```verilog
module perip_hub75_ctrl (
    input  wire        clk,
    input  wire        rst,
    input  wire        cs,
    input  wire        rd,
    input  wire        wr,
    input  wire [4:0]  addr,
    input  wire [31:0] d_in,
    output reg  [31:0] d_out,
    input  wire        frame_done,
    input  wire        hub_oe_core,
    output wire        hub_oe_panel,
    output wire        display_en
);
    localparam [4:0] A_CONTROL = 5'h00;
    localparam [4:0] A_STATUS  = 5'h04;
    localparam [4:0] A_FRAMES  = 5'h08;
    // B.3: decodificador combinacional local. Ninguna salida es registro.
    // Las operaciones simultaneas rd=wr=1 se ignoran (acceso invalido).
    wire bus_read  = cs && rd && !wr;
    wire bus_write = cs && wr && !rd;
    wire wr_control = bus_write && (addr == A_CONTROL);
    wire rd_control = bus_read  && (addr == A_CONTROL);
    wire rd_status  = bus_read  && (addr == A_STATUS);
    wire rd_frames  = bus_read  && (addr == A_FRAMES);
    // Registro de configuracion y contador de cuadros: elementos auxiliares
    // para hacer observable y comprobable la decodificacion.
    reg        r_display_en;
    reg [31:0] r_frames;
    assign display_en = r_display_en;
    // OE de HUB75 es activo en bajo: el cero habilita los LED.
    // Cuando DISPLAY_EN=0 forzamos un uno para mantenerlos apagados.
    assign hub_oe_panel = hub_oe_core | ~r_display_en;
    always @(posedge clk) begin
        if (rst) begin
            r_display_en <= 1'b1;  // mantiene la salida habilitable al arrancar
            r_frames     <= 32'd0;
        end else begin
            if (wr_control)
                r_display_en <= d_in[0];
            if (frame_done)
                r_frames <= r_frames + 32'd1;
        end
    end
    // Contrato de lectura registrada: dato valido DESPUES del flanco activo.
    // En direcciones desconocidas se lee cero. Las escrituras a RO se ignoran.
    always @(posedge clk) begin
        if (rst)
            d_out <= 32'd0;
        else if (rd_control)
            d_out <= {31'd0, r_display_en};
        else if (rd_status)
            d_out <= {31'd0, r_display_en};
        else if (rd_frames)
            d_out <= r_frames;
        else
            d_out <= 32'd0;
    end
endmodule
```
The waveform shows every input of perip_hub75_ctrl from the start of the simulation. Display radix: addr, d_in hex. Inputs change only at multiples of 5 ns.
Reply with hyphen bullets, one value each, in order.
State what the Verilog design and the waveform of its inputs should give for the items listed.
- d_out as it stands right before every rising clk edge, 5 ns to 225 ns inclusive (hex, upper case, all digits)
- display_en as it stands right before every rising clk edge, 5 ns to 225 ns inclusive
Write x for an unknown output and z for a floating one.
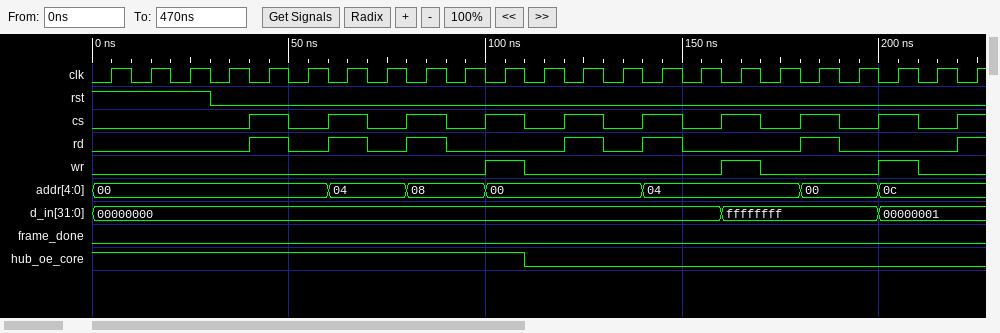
- x, 00000000, 00000000, 00000000, 00000000, 00000001, 00000000, 00000001, 00000000, 00000000, 00000000, 00000000, 00000000, 00000000, 00000000, 00000000, 00000000, 00000000, 00000000, 00000000, 00000000, 00000000, 00000000
- x 1 1 1 1 1 1 1 1 1 1 0 0 0 0 0 0 0 0 0 0 0 0
